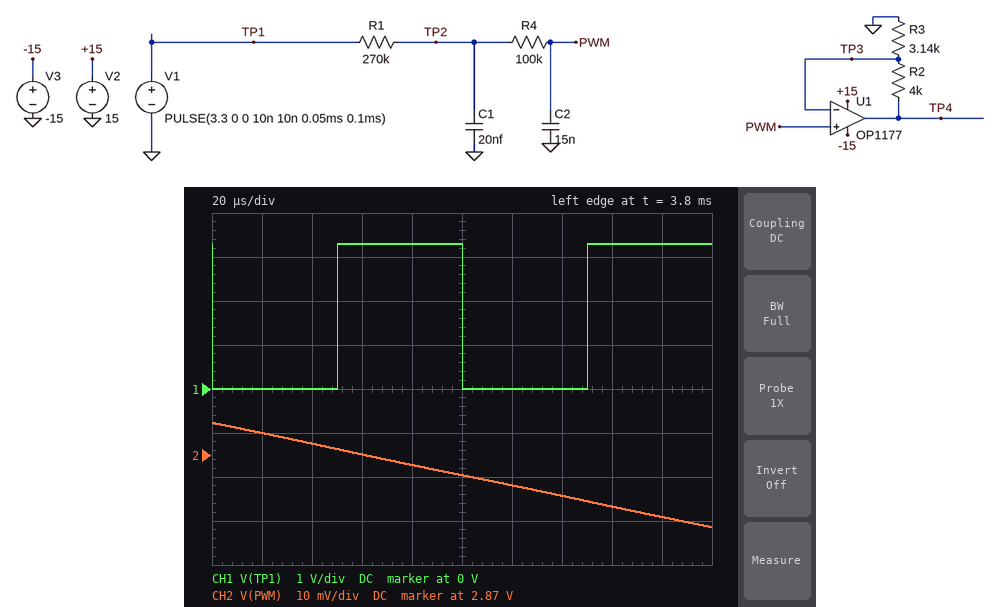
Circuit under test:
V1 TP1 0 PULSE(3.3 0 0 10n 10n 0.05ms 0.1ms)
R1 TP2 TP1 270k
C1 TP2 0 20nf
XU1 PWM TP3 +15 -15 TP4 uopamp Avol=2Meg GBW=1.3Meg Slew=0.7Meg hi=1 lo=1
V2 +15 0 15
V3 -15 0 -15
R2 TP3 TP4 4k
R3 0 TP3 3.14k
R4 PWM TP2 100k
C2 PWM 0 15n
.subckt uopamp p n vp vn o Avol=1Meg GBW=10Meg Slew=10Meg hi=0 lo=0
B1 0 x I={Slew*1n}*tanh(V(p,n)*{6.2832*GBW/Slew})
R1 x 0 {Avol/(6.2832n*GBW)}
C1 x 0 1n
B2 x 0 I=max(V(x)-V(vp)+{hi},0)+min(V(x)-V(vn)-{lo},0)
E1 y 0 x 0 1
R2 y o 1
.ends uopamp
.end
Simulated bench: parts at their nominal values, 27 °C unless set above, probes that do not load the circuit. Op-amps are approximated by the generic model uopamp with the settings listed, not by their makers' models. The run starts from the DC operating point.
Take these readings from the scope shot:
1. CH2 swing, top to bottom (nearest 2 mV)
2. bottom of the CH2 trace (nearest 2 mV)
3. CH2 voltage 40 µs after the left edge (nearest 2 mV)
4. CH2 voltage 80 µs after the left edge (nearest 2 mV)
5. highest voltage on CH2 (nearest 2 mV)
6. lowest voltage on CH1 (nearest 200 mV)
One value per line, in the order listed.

24 mV
2.854 V
2.872 V
2.868 V
2.878 V
0 V
